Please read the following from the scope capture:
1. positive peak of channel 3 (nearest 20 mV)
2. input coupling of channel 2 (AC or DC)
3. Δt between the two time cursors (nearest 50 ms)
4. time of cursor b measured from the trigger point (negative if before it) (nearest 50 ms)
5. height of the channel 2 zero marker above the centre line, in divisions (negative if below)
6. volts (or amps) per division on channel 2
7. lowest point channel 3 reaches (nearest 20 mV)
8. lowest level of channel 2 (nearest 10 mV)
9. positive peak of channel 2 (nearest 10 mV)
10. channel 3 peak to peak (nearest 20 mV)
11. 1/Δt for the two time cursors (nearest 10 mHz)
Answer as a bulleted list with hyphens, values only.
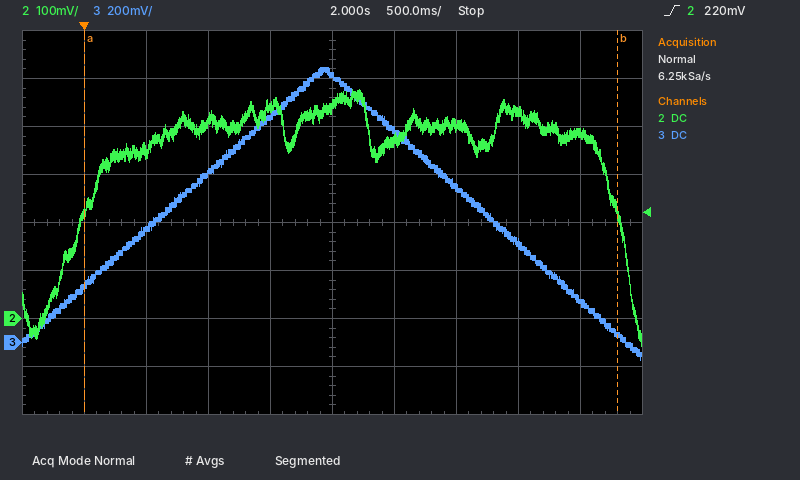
- 1.14 V
- DC
- 4.30 s
- +4.30 s
- -2.0 div
- 100 mV
- -80 mV
- -60 mV
- 480 mV
- 1.22 V
- 230 mHz
